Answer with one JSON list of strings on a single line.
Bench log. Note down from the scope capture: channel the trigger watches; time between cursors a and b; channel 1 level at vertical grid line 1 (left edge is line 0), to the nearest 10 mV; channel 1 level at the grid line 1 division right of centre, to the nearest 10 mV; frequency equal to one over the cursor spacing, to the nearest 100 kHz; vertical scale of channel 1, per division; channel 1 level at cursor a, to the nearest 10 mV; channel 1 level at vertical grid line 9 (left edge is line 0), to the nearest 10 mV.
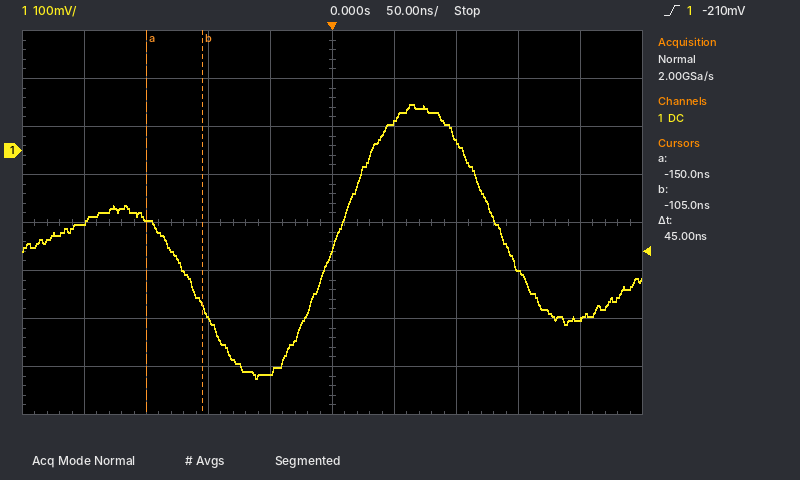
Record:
["channel 1", "45 ns", "-150 mV", "60 mV", "22.2 MHz", "100 mV", "-140 mV", "-350 mV"]
